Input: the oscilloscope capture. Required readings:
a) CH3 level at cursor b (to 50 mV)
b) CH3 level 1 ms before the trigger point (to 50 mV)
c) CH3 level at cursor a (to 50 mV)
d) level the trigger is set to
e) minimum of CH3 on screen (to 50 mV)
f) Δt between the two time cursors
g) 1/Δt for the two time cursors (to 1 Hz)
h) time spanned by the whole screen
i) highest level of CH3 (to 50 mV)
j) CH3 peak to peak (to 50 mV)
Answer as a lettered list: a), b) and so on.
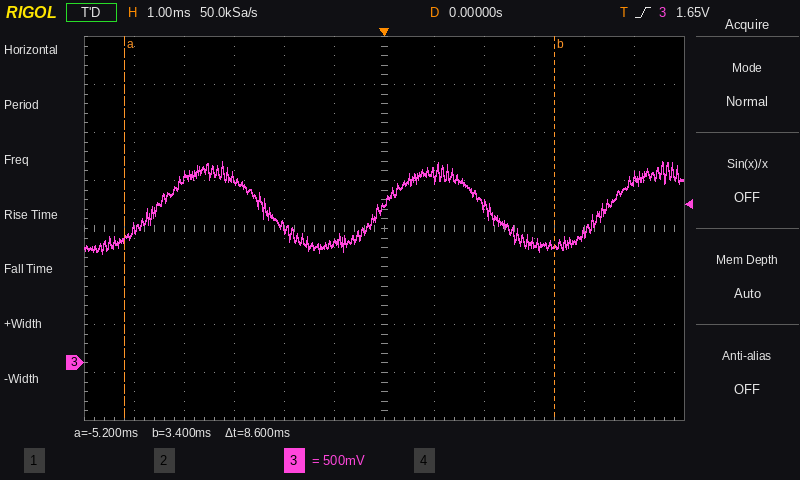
a) 1.20 V
b) 1.25 V
c) 1.30 V
d) 1.65 V
e) 1.15 V
f) 8.6 ms
g) 116 Hz
h) 12 ms
i) 2.10 V
j) 950 mV
